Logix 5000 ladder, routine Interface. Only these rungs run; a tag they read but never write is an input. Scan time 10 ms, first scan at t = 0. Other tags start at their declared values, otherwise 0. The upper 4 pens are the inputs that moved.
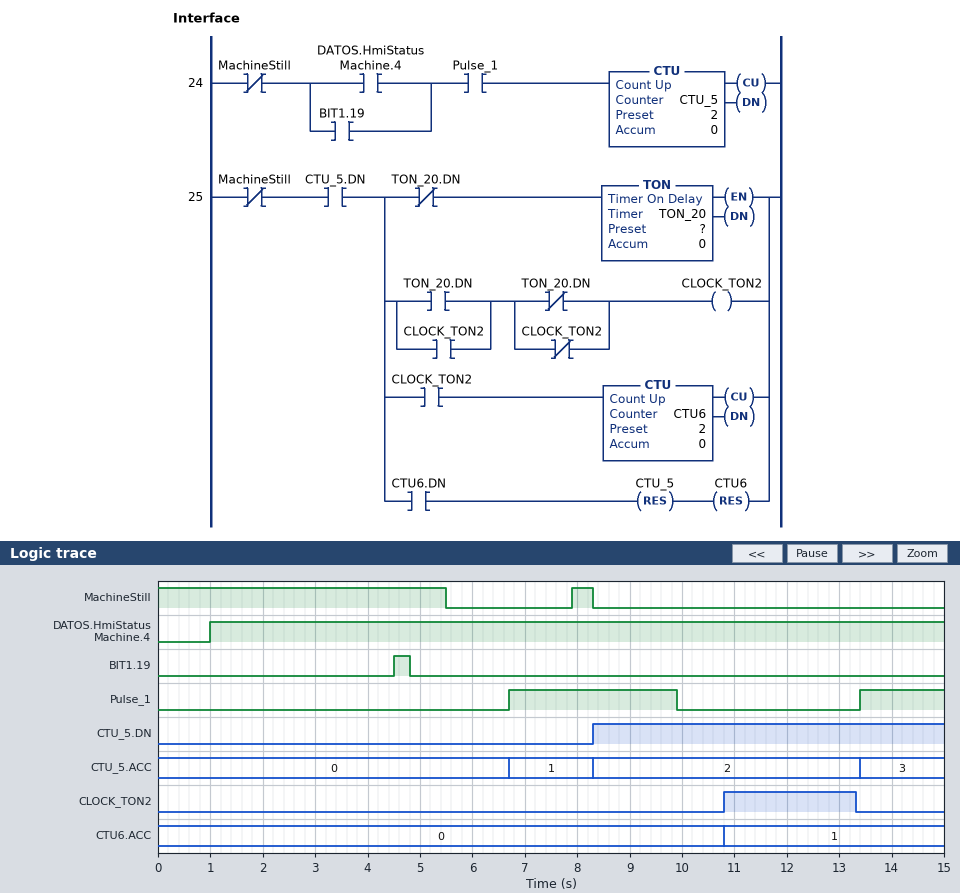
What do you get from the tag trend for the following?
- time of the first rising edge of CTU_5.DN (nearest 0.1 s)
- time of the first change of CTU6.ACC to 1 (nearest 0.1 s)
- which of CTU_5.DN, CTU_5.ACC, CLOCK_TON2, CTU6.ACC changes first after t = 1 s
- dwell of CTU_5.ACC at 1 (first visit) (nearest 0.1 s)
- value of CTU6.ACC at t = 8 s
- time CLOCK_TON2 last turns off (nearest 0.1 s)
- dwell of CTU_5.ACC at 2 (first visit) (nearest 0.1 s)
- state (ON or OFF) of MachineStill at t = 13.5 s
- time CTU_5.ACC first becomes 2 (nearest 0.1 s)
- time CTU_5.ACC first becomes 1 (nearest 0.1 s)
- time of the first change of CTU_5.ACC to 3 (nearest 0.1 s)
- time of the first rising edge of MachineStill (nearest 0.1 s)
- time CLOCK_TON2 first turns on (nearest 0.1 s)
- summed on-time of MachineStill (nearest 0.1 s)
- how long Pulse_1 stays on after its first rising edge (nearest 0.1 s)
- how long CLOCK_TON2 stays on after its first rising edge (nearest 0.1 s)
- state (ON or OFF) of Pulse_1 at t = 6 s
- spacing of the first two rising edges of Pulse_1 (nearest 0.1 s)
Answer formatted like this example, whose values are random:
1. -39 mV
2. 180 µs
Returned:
1. 8.3 s
2. 10.8 s
3. CTU_5.ACC
4. 1.6 s
5. 0
6. 13.3 s
7. 5.1 s
8. OFF
9. 8.3 s
10. 6.7 s
11. 13.4 s
12. 7.9 s
13. 10.8 s
14. 5.9 s
15. 3.2 s
16. 2.5 s
17. OFF
18. 6.7 s
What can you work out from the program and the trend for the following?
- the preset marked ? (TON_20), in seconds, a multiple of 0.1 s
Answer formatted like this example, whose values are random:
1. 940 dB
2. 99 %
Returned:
1. 2.5 s
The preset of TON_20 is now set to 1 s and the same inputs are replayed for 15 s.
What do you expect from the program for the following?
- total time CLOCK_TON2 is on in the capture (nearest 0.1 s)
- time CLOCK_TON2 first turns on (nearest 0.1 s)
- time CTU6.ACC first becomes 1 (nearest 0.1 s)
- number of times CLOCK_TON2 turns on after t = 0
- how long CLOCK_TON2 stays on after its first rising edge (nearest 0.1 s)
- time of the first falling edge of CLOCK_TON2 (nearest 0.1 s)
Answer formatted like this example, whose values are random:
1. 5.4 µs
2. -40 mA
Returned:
1. 1.0 s
2. 9.3 s
3. 9.3 s
4. 2
5. 1.0 s
6. 10.3 s
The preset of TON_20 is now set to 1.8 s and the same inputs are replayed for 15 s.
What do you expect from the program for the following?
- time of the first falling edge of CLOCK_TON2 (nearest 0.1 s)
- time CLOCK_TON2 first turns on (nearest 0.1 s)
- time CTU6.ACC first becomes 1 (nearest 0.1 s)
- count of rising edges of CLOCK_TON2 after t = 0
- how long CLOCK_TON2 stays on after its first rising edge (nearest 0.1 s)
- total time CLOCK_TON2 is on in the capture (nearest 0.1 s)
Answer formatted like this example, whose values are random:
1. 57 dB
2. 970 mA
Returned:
1. 11.9 s
2. 10.1 s
3. 10.1 s
4. 2
5. 1.8 s
6. 1.8 s
